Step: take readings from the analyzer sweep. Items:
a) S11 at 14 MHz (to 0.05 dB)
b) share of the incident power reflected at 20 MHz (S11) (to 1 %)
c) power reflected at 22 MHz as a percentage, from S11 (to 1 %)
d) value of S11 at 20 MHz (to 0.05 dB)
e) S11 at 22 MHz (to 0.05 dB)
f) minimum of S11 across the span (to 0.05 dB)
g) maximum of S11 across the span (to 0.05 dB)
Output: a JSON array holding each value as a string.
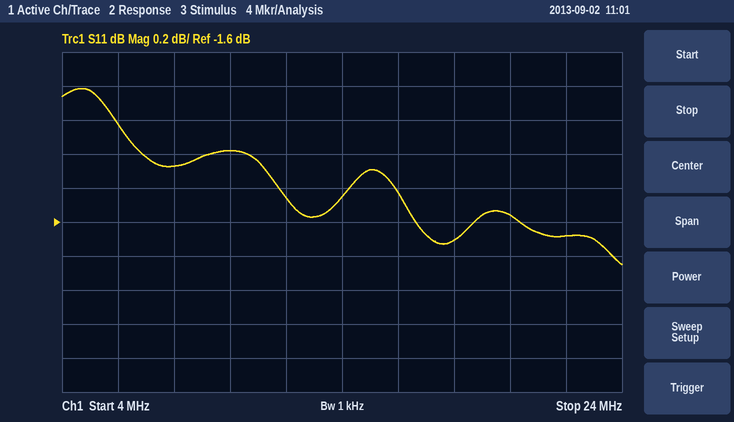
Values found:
["-1.45 dB", "70 %", "68 %", "-1.55 dB", "-1.70 dB", "-1.85 dB", "-0.80 dB"]
